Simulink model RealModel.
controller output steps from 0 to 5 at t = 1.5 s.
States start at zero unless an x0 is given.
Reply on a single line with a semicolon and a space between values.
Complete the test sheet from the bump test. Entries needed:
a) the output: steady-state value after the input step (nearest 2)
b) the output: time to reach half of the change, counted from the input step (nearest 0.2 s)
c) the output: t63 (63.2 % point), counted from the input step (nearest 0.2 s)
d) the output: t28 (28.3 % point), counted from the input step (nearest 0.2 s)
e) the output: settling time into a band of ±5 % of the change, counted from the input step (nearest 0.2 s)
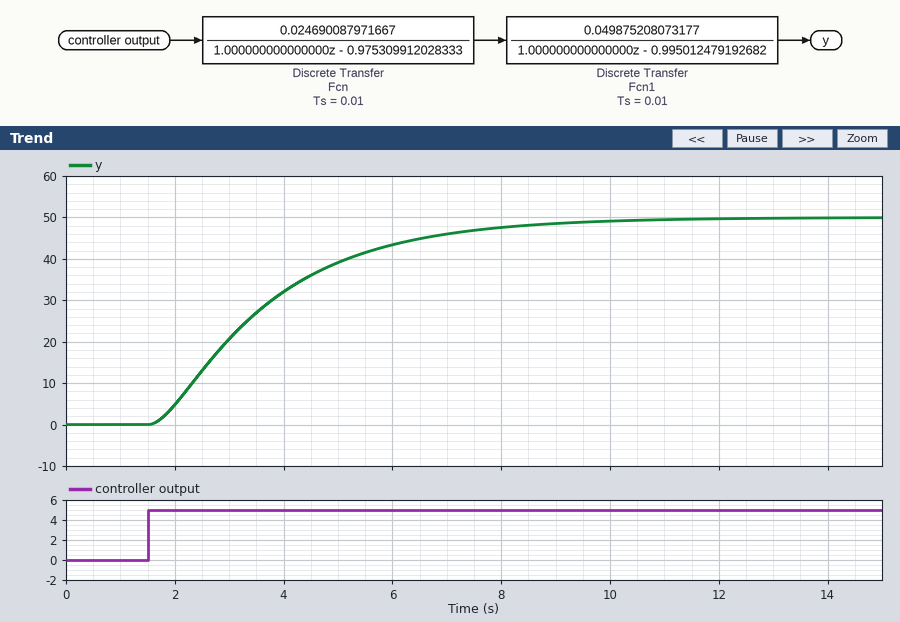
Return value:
50; 1.8 s; 2.4 s; 1.0 s; 6.4 s
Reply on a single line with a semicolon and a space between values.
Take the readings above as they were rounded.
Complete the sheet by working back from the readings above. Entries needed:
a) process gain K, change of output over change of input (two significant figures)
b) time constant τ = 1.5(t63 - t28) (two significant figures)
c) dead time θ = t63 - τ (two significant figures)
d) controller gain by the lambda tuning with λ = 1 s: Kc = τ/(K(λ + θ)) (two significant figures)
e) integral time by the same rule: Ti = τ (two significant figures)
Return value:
10; 2.1 s; 0.30 s; 0.16; 2.1 s
